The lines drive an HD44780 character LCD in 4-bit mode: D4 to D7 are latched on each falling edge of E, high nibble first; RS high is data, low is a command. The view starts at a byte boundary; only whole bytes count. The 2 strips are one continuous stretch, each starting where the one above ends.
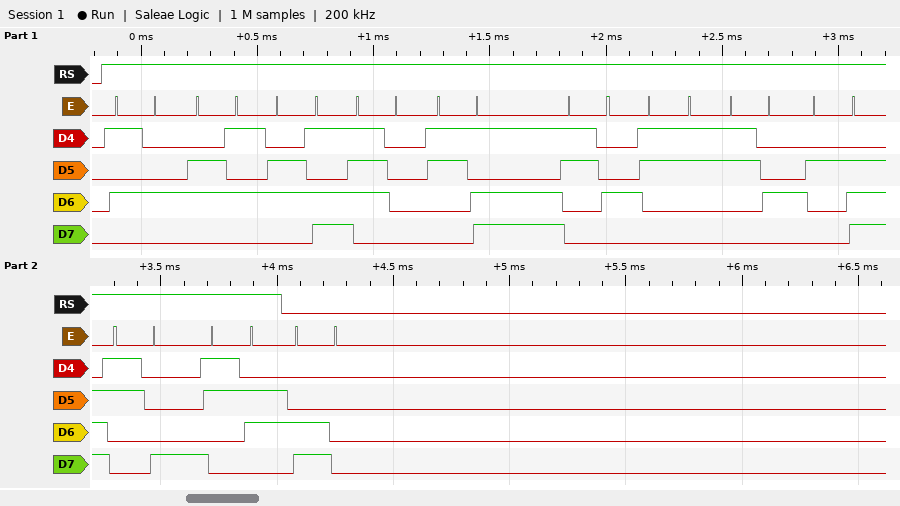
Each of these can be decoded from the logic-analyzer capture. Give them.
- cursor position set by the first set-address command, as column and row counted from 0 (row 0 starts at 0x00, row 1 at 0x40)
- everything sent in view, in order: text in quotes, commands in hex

column 0, row 1
"Temp=434.86" 0xC0
